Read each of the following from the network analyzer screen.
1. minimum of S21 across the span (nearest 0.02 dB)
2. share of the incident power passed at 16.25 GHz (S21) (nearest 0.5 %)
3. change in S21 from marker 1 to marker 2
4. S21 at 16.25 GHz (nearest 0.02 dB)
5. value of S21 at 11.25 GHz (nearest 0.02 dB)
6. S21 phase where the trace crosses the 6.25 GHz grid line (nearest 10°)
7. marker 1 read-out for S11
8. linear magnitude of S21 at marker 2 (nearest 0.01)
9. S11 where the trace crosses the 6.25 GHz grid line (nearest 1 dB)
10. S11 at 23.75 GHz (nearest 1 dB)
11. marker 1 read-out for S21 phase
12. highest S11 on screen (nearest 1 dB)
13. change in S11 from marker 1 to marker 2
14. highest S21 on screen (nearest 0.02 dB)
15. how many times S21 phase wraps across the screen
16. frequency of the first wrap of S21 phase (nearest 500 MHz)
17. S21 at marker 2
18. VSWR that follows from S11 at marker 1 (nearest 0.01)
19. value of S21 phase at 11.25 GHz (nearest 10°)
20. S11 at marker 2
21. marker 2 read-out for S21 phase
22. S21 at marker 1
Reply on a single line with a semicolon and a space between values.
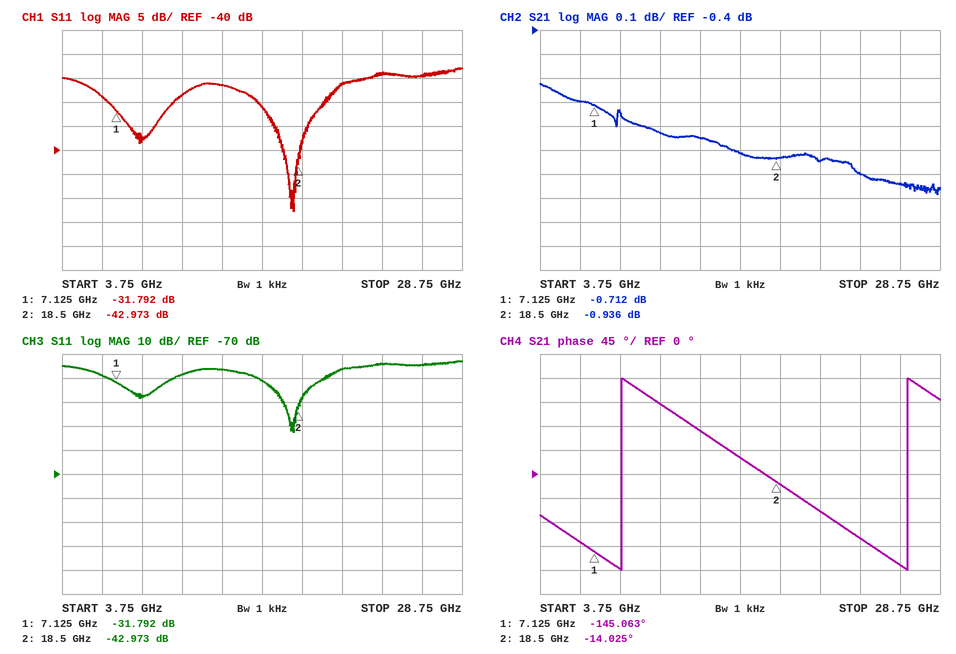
-1.08 dB; 81.0 %; -0.224 dB; -0.92 dB; -0.82 dB; -130°; -31.792 dB; 0.90; -29 dB; -24 dB; -145.063°; -23 dB; -11.181 dB; -0.62 dB; 2; 9.0 GHz; -0.936 dB; 1.05; 130°; -42.973 dB; -14.025°; -0.712 dB
